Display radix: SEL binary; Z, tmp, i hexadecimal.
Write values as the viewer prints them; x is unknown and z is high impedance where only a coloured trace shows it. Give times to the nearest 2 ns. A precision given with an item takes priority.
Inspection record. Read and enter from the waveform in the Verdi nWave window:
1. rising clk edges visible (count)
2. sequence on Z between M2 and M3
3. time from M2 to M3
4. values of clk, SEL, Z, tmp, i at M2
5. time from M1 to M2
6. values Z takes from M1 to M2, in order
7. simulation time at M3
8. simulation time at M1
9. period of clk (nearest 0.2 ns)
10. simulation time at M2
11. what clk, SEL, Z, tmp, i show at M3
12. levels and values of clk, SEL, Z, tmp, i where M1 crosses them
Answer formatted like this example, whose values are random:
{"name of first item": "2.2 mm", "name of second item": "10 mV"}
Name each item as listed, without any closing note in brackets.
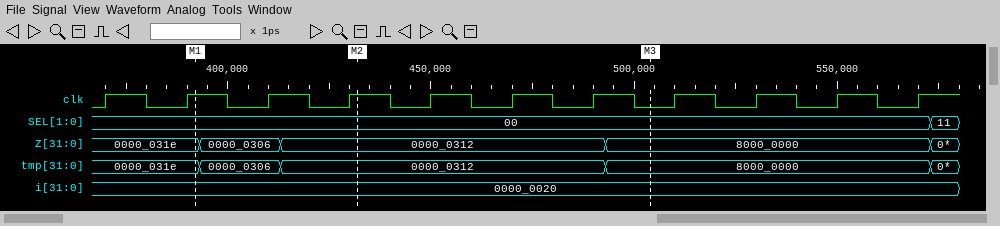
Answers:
{"rising clk edges visible": "11", "sequence on Z between M2 and M3": "0000_0312, 8000_0000", "time from M2 to M3": "72 ns", "values of clk, SEL, Z, tmp, i at M2": "clk=1, SEL=00, Z=0000_0312, tmp=0000_0312, i=0000_0020", "time from M1 to M2": "40 ns", "values Z takes from M1 to M2, in order": "0000_031e, 0000_0306, 0000_0312", "simulation time at M3": "504 ns", "simulation time at M1": "392 ns", "period of clk": "20 ns", "simulation time at M2": "432 ns", "what clk, SEL, Z, tmp, i show at M3": "clk=0, SEL=00, Z=8000_0000, tmp=8000_0000, i=0000_0020", "levels and values of clk, SEL, Z, tmp, i where M1 crosses them": "clk=1, SEL=00, Z=0000_031e, tmp=0000_031e, i=0000_0020"}
